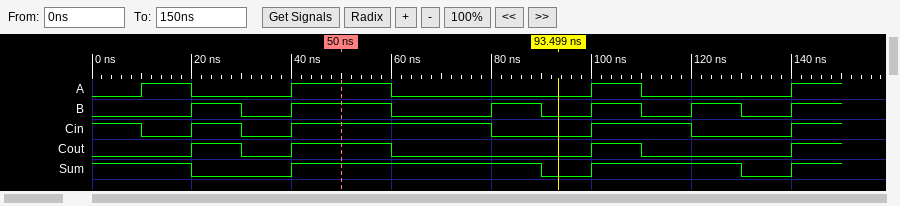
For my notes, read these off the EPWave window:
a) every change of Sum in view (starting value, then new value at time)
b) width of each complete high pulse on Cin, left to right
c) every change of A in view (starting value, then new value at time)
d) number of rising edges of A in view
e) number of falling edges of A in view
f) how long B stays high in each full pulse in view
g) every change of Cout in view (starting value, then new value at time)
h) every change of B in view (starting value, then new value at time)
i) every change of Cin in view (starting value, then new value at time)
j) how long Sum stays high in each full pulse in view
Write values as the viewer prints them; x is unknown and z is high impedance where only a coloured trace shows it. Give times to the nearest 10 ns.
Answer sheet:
1, 0 at 20 ns, 1 at 40 ns, 0 at 90 ns, 1 at 100 ns, 0 at 130 ns, 1 at 140 ns
10 ns, 40 ns, 20 ns
0, 1 at 10 ns, 0 at 20 ns, 1 at 40 ns, 0 at 60 ns, 1 at 100 ns, 0 at 110 ns, 1 at 140 ns
4
3
10 ns, 20 ns, 10 ns, 10 ns, 10 ns
0, 1 at 20 ns, 0 at 30 ns, 1 at 40 ns, 0 at 60 ns, 1 at 100 ns, 0 at 110 ns, 1 at 140 ns
0, 1 at 20 ns, 0 at 30 ns, 1 at 40 ns, 0 at 60 ns, 1 at 80 ns, 0 at 90 ns, 1 at 100 ns, 0 at 110 ns, 1 at 120 ns, 0 at 130 ns, 1 at 140 ns
1, 0 at 10 ns, 1 at 20 ns, 0 at 30 ns, 1 at 40 ns, 0 at 80 ns, 1 at 100 ns, 0 at 120 ns, 1 at 140 ns
50 ns, 30 ns
